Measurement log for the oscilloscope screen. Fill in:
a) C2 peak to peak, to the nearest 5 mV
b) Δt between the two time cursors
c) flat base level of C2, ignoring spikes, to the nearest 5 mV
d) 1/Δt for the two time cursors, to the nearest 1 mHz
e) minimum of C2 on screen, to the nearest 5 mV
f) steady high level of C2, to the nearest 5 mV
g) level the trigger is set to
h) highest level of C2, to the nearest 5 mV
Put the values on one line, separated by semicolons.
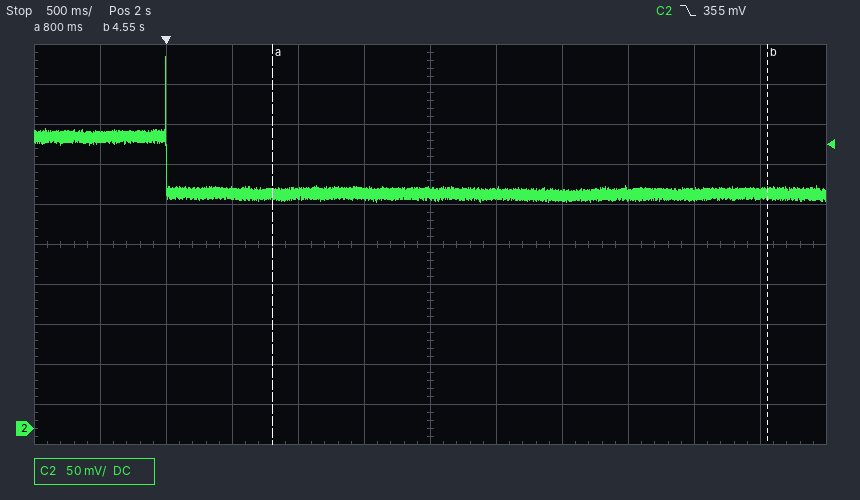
180 mV; 3.75 s; 295 mV; 267 mHz; 285 mV; 365 mV; 355 mV; 465 mV
